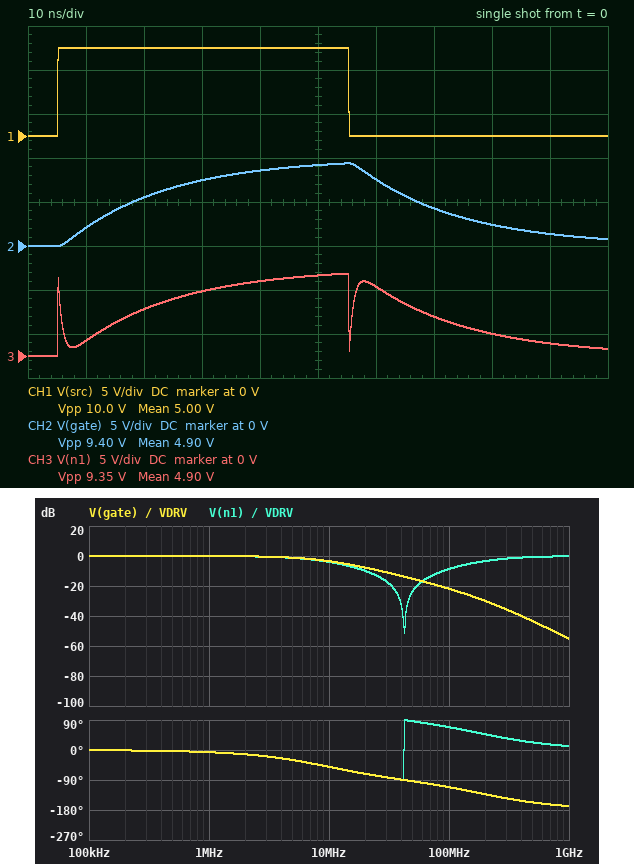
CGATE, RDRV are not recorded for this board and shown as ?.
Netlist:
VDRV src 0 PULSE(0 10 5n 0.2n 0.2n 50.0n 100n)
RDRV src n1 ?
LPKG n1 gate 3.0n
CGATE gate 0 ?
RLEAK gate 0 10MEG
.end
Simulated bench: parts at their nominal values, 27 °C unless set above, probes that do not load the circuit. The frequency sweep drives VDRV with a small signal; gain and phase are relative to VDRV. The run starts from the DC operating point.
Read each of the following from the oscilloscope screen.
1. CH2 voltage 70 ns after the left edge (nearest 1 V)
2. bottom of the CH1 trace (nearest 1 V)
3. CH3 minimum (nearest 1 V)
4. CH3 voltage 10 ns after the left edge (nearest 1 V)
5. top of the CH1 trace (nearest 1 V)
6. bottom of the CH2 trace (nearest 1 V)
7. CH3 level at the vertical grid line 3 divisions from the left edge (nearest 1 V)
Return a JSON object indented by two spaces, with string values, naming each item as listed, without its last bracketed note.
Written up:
{
  "CH2 voltage 70 ns after the left edge": "4 V",
  "bottom of the CH1 trace": "0 V",
  "CH3 minimum": "0 V",
  "CH3 voltage 10 ns after the left edge": "2 V",
  "top of the CH1 trace": "10 V",
  "bottom of the CH2 trace": "0 V",
  "CH3 level at the vertical grid line 3 divisions from the left edge": "7 V"
}
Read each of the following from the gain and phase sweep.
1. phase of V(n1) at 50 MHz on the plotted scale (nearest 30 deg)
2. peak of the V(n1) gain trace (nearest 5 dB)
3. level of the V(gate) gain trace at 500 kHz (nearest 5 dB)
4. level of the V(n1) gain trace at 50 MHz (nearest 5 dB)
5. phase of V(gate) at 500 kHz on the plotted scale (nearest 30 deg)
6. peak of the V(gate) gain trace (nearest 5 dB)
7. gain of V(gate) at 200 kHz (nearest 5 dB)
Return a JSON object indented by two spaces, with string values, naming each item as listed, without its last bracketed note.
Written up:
{
  "phase of V(n1) at 50 MHz on the plotted scale": "90 deg",
  "peak of the V(n1) gain trace": "0 dB",
  "level of the V(gate) gain trace at 500 kHz": "0 dB",
  "level of the V(n1) gain trace at 50 MHz": "-25 dB",
  "phase of V(gate) at 500 kHz on the plotted scale": "0 deg",
  "peak of the V(gate) gain trace": "0 dB",
  "gain of V(gate) at 200 kHz": "0 dB"
}
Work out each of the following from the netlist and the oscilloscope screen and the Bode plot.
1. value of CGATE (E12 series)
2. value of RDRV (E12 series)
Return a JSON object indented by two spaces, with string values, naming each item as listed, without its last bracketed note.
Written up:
{
  "value of CGATE": "4.7 nF",
  "value of RDRV": "3.9 Ω"
}
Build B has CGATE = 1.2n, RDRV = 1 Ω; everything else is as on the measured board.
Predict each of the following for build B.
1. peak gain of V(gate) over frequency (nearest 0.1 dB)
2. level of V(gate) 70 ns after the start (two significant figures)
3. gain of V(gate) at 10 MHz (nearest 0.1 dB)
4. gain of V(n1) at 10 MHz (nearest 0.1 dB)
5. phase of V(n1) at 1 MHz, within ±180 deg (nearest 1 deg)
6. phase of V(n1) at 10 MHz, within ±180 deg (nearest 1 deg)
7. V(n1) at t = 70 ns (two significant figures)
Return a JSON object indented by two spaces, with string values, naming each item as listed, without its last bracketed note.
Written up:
{
  "peak gain of V(gate) over frequency": "4.4 dB",
  "level of V(gate) 70 ns after the start": "670 mV",
  "gain of V(gate) at 10 MHz": "0.1 dB",
  "gain of V(n1) at 10 MHz": "0 dB",
  "phase of V(n1) at 1 MHz, within ±180 deg": "0 deg",
  "phase of V(n1) at 10 MHz, within ±180 deg": "-4 deg",
  "V(n1) at t = 70 ns": "500 mV"
}
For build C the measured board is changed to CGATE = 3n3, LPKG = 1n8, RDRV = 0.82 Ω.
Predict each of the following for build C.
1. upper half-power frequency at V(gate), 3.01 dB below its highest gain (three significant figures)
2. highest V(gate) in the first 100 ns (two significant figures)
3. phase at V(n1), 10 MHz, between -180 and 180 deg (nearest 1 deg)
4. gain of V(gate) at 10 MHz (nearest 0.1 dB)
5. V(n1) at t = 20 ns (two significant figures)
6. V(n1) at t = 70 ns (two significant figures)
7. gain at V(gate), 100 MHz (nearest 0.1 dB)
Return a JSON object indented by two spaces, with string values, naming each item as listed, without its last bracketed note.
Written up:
{
  "upper half-power frequency at V(gate), 3.01 dB below its highest gain": "74.7 MHz",
  "highest V(gate) in the first 100 ns": "11 V",
  "phase at V(n1), 10 MHz, between -180 and 180 deg": "-10 deg",
  "gain of V(gate) at 10 MHz": "0.1 dB",
  "V(n1) at t = 20 ns": "10 V",
  "V(n1) at t = 70 ns": "-450 mV",
  "gain at V(gate), 100 MHz": "-6.7 dB"
}
